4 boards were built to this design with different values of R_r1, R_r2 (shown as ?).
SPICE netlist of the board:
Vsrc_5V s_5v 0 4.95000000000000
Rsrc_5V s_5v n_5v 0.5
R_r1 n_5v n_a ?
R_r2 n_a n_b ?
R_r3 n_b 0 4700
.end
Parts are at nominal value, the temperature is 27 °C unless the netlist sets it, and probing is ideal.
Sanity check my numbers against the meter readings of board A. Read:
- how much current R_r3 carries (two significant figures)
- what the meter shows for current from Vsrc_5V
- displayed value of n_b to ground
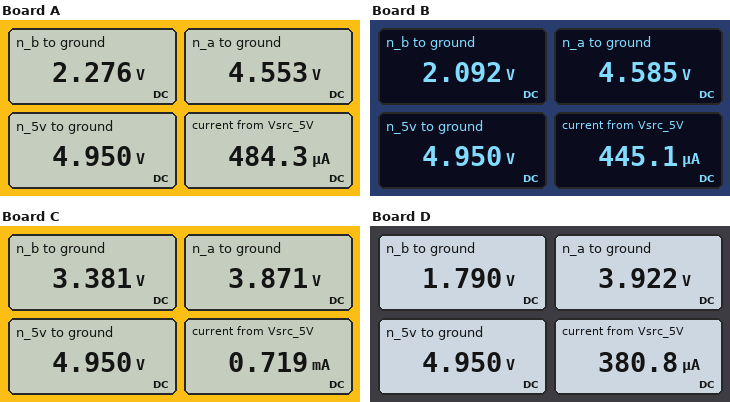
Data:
480 µA
484.3 µA
2.276 V
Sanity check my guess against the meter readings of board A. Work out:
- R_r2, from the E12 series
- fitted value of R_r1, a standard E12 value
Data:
4.7 kΩ
820 Ω
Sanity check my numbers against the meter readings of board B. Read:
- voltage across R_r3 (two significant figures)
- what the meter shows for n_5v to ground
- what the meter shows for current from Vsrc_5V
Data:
2.1 V
4.950 V
445.1 µA
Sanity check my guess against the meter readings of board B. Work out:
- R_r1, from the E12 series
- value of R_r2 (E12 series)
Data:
820 Ω
5.6 kΩ
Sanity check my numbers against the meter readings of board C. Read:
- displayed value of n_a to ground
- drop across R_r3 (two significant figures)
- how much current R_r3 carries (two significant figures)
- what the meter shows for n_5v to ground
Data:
3.871 V
3.4 V
720 µA
4.950 V
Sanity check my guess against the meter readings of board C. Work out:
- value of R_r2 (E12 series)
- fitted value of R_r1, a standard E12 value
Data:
680 Ω
1.5 kΩ
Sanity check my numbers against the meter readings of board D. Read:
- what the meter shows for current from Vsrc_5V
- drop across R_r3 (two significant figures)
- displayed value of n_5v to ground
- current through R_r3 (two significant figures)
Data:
380.8 µA
1.8 V
4.950 V
380 µA
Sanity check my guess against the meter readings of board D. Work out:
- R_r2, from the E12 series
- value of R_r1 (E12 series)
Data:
5.6 kΩ
2.7 kΩ
